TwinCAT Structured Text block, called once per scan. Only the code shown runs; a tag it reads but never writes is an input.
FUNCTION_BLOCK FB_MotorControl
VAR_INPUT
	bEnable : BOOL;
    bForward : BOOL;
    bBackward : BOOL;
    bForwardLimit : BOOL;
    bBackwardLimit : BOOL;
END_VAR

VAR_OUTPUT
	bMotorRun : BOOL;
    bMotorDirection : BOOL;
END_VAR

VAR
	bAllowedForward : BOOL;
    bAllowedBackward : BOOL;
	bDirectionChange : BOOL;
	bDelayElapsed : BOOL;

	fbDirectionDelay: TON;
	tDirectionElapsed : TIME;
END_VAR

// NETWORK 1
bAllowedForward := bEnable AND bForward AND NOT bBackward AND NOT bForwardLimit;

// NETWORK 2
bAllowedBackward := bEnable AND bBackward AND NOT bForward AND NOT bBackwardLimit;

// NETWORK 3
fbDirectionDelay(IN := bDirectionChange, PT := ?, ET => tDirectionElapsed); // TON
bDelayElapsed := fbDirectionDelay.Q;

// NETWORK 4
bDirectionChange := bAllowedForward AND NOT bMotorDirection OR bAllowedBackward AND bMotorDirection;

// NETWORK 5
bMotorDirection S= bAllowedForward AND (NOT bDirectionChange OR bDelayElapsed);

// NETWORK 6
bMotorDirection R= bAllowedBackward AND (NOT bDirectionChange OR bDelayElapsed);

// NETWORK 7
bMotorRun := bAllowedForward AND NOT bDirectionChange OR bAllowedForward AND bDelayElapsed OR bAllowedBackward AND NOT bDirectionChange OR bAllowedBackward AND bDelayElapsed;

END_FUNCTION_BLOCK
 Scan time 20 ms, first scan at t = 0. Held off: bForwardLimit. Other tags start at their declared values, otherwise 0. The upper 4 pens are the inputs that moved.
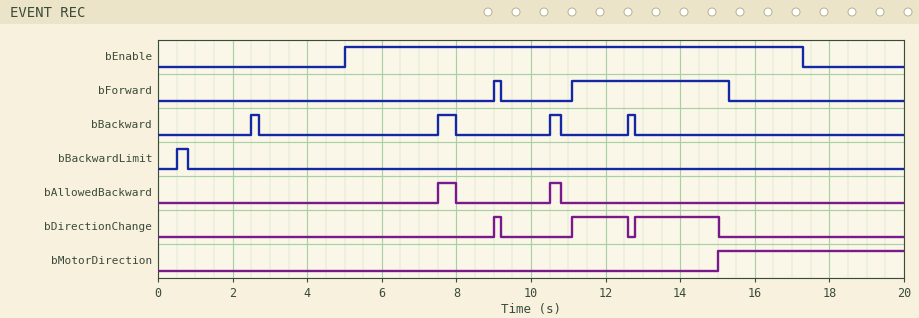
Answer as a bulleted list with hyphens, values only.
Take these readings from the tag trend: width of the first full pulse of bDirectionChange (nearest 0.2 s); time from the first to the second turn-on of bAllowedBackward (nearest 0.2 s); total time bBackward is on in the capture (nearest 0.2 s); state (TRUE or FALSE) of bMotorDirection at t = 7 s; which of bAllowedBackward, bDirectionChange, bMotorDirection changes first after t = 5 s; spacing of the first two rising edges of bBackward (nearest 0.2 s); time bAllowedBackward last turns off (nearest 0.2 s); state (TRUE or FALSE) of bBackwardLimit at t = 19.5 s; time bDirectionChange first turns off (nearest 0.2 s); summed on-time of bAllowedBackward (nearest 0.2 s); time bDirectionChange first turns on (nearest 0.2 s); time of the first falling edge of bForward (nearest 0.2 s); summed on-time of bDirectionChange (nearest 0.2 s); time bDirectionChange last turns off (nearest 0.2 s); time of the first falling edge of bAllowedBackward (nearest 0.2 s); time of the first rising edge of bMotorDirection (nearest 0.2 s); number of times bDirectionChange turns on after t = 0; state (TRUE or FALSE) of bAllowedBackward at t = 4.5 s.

- 0.2 s
- 3.0 s
- 1.2 s
- FALSE
- bAllowedBackward
- 5.0 s
- 10.8 s
- FALSE
- 9.2 s
- 0.8 s
- 9.0 s
- 9.2 s
- 4.0 s
- 15.0 s
- 8.0 s
- 15.0 s
- 3
- FALSE
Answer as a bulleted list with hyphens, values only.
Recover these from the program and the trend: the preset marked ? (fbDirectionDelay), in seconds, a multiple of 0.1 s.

- 2.2 s
